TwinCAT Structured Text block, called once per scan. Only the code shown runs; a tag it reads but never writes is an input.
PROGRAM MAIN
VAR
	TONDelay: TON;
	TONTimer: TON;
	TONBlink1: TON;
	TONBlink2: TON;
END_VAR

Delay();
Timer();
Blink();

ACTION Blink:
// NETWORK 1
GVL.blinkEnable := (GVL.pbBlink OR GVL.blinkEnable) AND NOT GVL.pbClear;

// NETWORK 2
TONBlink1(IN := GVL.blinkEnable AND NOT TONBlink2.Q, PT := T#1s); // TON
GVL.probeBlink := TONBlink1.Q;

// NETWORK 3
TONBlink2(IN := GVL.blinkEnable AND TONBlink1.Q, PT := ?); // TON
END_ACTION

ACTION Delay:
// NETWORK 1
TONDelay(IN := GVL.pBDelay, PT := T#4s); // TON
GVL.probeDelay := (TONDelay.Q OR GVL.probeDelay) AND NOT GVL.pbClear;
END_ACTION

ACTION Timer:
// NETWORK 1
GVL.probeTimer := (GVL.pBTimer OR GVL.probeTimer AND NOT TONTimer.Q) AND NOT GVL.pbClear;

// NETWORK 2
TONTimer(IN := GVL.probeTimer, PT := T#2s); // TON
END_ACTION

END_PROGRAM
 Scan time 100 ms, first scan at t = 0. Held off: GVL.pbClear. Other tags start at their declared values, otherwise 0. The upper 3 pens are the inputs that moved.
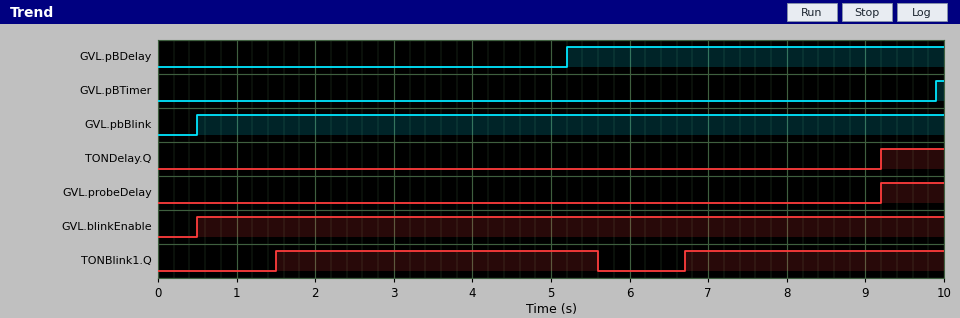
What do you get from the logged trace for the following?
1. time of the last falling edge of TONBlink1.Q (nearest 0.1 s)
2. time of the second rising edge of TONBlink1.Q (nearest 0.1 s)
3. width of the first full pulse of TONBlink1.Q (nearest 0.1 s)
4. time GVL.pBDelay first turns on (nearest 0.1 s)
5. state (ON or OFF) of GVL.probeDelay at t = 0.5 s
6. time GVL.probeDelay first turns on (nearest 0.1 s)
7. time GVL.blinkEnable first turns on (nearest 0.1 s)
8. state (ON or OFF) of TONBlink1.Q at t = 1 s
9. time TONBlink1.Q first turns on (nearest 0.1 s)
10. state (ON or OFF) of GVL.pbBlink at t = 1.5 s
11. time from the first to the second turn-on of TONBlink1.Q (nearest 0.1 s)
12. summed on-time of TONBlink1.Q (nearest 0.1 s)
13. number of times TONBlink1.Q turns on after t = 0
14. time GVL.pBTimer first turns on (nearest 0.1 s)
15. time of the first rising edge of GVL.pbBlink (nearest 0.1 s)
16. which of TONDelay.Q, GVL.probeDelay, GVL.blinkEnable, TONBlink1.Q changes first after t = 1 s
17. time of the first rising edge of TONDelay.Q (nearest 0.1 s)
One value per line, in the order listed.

5.6 s
6.7 s
4.1 s
5.2 s
OFF
9.2 s
0.5 s
OFF
1.5 s
ON
5.2 s
7.4 s
2
9.9 s
0.5 s
TONBlink1.Q
9.2 s
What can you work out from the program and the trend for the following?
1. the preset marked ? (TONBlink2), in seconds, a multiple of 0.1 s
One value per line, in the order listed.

4.0 s
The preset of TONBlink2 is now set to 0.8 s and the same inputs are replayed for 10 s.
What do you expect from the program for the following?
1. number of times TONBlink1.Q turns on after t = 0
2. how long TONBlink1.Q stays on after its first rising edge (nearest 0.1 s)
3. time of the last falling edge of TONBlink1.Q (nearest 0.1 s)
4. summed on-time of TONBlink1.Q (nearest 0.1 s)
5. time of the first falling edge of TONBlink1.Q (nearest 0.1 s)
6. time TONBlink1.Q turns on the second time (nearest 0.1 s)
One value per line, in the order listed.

5
0.9 s
8.4 s
4.1 s
2.4 s
3.5 s
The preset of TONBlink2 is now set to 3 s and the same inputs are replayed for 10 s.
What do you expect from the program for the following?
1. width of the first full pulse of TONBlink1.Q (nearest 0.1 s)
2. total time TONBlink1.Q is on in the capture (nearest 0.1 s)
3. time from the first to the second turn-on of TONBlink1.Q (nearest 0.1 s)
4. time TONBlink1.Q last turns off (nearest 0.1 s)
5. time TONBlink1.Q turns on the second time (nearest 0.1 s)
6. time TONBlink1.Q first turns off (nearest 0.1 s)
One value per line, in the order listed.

3.1 s
6.3 s
4.2 s
8.8 s
5.7 s
4.6 s
